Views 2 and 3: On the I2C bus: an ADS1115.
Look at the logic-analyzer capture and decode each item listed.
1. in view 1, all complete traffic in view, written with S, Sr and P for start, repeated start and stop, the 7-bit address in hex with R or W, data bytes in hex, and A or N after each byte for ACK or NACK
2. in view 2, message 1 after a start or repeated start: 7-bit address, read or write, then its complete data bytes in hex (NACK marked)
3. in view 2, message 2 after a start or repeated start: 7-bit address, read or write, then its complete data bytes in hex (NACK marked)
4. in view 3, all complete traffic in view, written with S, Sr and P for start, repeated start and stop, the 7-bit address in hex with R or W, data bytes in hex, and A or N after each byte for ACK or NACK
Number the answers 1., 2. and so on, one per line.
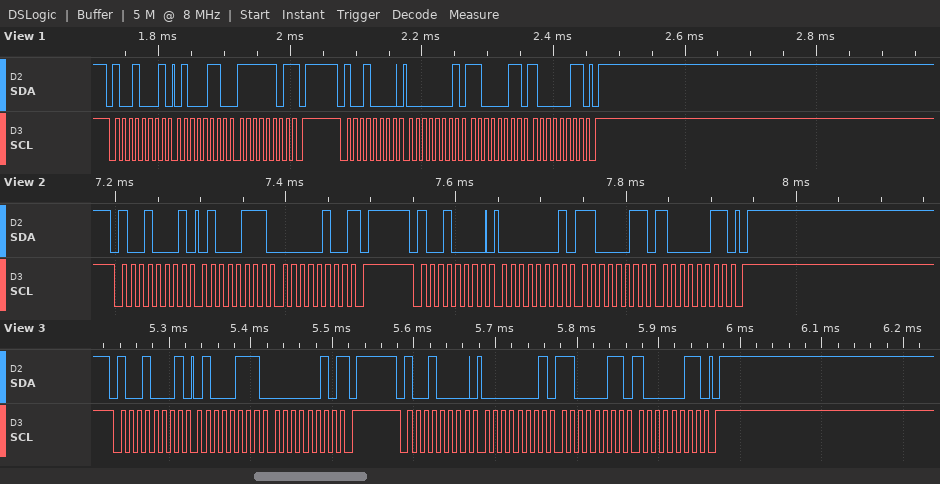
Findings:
1. S 48R A 46 A FD N P S 48W A 01 A C3 A 83 A P
2. 0x48 read: 47 04 NACK
3. 0x48 write: 01 C3 83
4. S 48R A 47 A 02 N P S 48W A 01 A C3 A 83 A P
